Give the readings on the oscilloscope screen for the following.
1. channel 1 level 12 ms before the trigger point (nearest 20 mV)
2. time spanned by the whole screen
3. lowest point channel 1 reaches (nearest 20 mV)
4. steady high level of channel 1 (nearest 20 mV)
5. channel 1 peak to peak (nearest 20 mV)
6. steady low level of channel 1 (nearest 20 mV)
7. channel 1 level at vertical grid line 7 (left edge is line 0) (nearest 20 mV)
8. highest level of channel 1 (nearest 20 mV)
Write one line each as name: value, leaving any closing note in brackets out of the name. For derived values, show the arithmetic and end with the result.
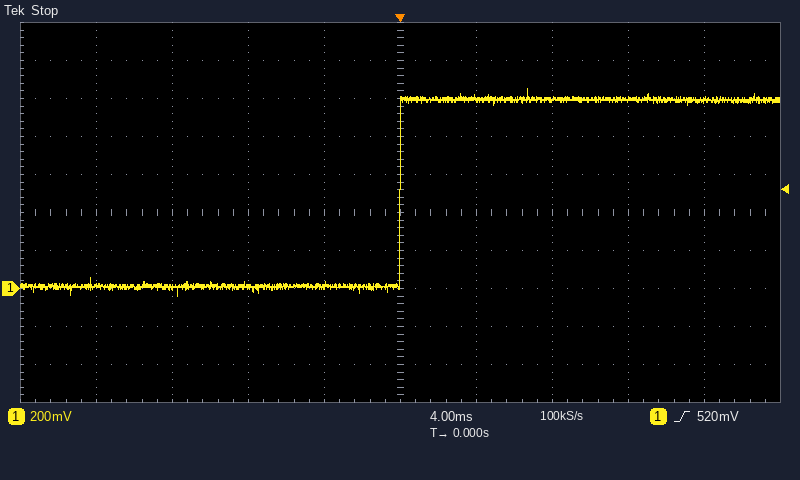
channel 1 level 12 ms before the trigger point: 0 mV
time spanned by the whole screen: 40 ms
lowest point channel 1 reaches: -40 mV
steady high level of channel 1: 1.00 V
channel 1 peak to peak: 1.06 V − (-40 mV) = 1.10 V
steady low level of channel 1: 20 mV
channel 1 level at vertical grid line 7 (left edge is line 0): 1.00 V
highest level of channel 1: 1.06 V
